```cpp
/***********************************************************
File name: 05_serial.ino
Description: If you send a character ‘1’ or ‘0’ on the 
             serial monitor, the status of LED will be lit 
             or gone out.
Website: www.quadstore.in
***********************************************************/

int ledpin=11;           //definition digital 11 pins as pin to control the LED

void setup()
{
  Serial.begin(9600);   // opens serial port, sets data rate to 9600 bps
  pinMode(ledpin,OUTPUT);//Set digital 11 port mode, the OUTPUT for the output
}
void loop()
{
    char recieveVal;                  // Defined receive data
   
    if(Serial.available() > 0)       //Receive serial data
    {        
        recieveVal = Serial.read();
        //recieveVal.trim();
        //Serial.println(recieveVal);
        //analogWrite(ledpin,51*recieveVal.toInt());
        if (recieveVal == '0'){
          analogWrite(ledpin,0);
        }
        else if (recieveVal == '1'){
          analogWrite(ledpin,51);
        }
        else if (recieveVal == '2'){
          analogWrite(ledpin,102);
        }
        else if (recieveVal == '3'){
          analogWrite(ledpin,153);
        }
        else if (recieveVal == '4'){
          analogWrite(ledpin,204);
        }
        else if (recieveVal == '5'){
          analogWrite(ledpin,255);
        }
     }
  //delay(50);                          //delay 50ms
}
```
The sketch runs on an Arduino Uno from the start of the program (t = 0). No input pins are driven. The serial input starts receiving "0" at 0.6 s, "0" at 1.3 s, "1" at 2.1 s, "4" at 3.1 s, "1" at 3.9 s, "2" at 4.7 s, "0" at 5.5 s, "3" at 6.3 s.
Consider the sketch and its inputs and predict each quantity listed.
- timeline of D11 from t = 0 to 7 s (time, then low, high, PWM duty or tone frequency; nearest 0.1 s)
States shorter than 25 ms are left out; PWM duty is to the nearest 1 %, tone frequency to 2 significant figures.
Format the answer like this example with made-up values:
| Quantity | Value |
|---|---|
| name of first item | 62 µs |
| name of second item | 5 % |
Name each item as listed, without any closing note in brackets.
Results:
| Quantity | Value |
|---|---|
| timeline of D11 from t = 0 to 7 s | 0 s low; 2.1 s PWM 20 %; 3.1 s PWM 80 %; 3.9 s PWM 20 %; 4.7 s PWM 40 %; 5.5 s low; 6.3 s PWM 60 % |
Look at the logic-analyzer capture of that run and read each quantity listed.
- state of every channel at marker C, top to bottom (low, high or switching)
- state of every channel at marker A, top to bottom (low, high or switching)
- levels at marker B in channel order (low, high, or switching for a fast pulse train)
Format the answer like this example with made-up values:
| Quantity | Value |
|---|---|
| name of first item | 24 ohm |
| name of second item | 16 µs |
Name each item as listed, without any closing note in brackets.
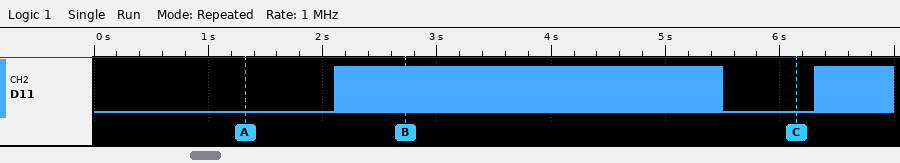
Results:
| Quantity | Value |
|---|---|
| state of every channel at marker C, top to bottom | D11 low |
| state of every channel at marker A, top to bottom | D11 low |
| levels at marker B in channel order | D11 switching |
